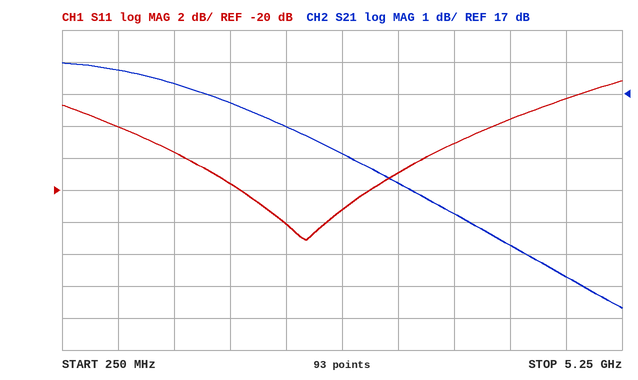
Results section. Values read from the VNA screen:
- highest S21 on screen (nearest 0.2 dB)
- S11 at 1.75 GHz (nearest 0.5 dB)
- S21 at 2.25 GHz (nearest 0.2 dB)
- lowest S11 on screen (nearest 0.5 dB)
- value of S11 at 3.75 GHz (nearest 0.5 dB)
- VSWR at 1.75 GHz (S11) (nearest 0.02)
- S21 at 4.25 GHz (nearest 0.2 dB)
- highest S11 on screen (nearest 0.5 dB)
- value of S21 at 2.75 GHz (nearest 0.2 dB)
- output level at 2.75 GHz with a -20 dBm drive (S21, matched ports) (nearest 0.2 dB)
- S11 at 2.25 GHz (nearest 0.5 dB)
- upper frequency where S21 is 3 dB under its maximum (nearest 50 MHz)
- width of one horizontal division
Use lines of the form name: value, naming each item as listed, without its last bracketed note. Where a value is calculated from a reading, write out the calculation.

highest S21 on screen: 18.0 dB
S11 at 1.75 GHz: -19.5 dB
S21 at 2.25 GHz: 16.0 dB
lowest S11 on screen: -23.0 dB
value of S11 at 3.75 GHz: -17.0 dB
VSWR at 1.75 GHz (S11): |Γ| = 10^(-19.5/20) = 0.1059; VSWR = (1 + 0.1059)/(1 − 0.1059) ≈ 1.24
S21 at 4.25 GHz: 12.2 dB
highest S11 on screen: -13.0 dB
value of S21 at 2.75 GHz: 15.2 dB
output level at 2.75 GHz with a -20 dBm drive (S21, matched ports): -20 dBm + (15.2 dB) = -4.8 dBm
S11 at 2.25 GHz: -22.0 dB
upper frequency where S21 is 3 dB under its maximum: 2.85 GHz
width of one horizontal division: 500 MHz
